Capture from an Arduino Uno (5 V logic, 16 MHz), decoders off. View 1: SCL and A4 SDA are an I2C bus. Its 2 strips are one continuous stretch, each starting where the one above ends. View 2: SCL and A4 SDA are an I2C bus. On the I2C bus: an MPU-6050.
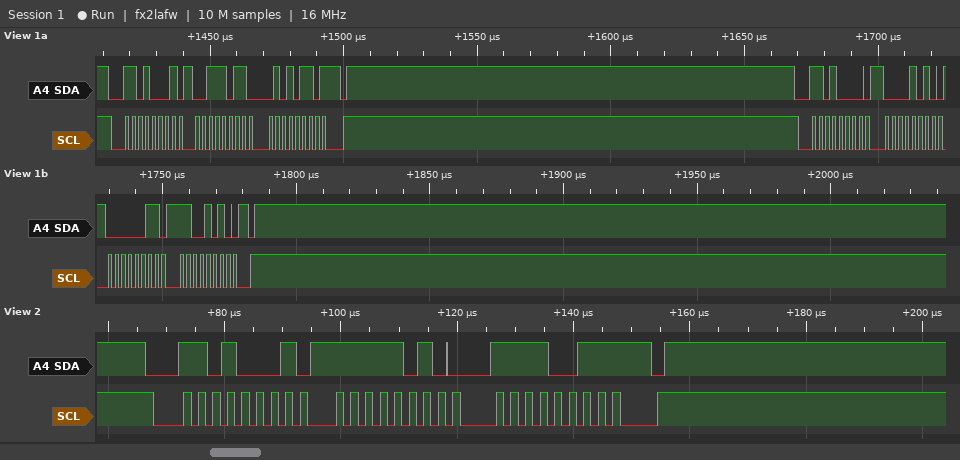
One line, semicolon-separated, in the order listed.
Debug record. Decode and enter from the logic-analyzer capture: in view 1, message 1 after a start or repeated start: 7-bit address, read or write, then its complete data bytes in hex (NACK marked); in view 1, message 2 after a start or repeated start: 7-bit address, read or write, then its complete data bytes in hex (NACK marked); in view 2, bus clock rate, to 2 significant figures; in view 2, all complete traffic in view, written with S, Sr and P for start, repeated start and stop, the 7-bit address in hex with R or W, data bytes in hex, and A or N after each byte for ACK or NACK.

0x68 read: 3B 56 NACK; 0x68 write: 0A 03 CA; 400 kHz; S 68R A FA A F3 N P
